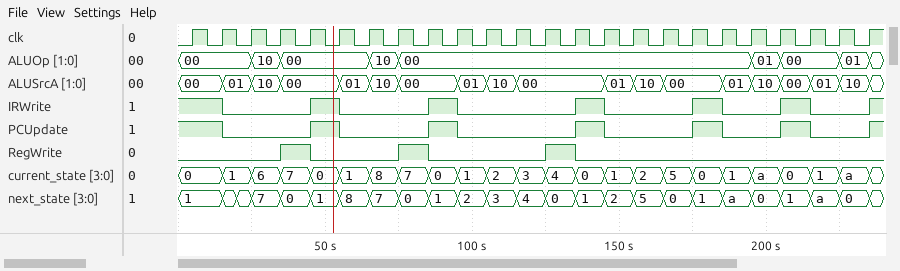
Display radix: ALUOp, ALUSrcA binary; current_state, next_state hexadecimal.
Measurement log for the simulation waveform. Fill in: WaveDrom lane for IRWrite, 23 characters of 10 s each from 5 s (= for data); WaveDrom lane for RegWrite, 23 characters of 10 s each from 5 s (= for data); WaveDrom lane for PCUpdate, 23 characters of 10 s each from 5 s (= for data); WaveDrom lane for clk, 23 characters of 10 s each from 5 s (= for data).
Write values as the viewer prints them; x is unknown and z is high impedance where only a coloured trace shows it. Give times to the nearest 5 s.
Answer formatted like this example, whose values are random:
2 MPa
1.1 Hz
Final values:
{name: 'IRWrite', wave: '10..10..10...10..10.10.'}
{name: 'RegWrite', wave: '0..10..10...10.........'}
{name: 'PCUpdate', wave: '10..10..10...10..10.10.'}
{name: 'clk', wave: 'p......................'}
